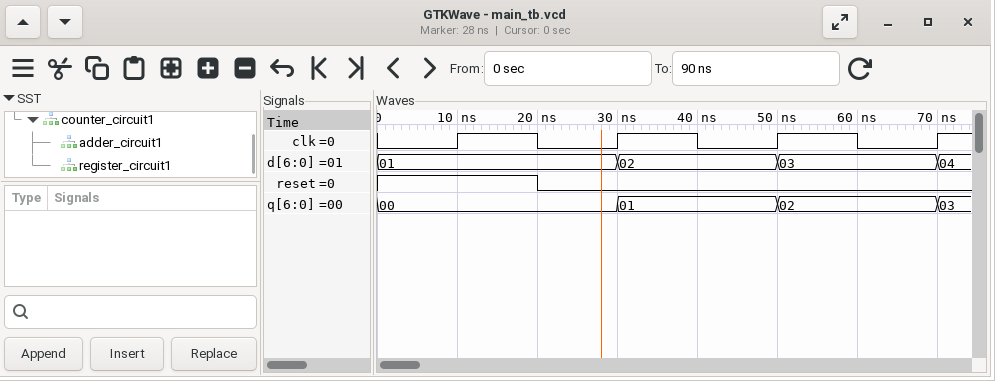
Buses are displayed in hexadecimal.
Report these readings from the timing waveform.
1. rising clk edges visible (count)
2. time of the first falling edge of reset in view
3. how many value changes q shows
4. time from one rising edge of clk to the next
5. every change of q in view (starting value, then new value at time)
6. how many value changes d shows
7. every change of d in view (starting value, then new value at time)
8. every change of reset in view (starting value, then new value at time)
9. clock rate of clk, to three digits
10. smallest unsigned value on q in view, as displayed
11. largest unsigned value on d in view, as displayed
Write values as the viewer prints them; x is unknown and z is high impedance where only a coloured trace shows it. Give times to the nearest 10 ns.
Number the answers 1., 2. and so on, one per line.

1. 4
2. 20 ns
3. 3
4. 20 ns
5. 00, 01 at 30 ns, 02 at 50 ns, 03 at 70 ns
6. 3
7. 01, 02 at 30 ns, 03 at 50 ns, 04 at 70 ns
8. 1, 0 at 20 ns
9. 50.0 MHz
10. 00
11. 04
